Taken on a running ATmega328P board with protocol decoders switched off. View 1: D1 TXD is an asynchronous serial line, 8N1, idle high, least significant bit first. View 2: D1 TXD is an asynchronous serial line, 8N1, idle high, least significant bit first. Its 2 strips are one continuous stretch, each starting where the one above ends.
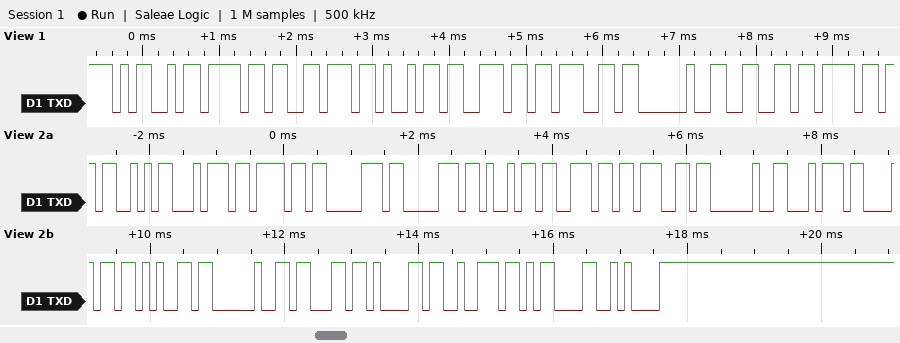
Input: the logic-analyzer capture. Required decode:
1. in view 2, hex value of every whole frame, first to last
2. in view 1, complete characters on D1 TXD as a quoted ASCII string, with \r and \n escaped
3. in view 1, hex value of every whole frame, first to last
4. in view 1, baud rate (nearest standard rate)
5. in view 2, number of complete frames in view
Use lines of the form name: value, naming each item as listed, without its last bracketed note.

in view 2, hex value of every whole frame, first to last: 53 74 6F 70 70 69 6E 67 20 74 68 65 20 63 61 72 0D 0A
in view 1, complete characters on D1 TXD as a quoted ASCII string, with \r and \n escaped: "Moving fo"
in view 1, hex value of every whole frame, first to last: 4D 6F 76 69 6E 67 20 66 6F
in view 1, baud rate: 9600 baud
in view 2, number of complete frames in view: 18
